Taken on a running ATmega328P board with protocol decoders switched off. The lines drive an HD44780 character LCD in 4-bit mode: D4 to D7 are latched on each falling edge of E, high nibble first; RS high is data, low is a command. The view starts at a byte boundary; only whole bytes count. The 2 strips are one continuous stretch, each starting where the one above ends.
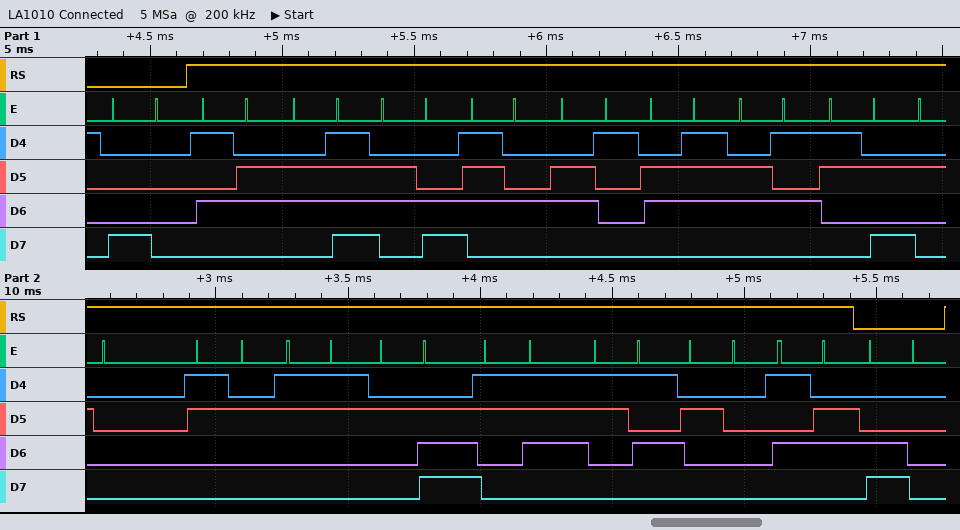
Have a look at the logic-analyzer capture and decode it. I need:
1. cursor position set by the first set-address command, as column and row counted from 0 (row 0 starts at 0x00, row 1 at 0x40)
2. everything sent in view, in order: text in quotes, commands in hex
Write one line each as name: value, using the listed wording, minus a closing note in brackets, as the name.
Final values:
cursor position set by the first set-address command, as column and row counted from 0: column 0, row 0
everything sent in view, in order: text in quotes, commands in hex: 0x80 "Voltage: 23.75 V" 0xC0
